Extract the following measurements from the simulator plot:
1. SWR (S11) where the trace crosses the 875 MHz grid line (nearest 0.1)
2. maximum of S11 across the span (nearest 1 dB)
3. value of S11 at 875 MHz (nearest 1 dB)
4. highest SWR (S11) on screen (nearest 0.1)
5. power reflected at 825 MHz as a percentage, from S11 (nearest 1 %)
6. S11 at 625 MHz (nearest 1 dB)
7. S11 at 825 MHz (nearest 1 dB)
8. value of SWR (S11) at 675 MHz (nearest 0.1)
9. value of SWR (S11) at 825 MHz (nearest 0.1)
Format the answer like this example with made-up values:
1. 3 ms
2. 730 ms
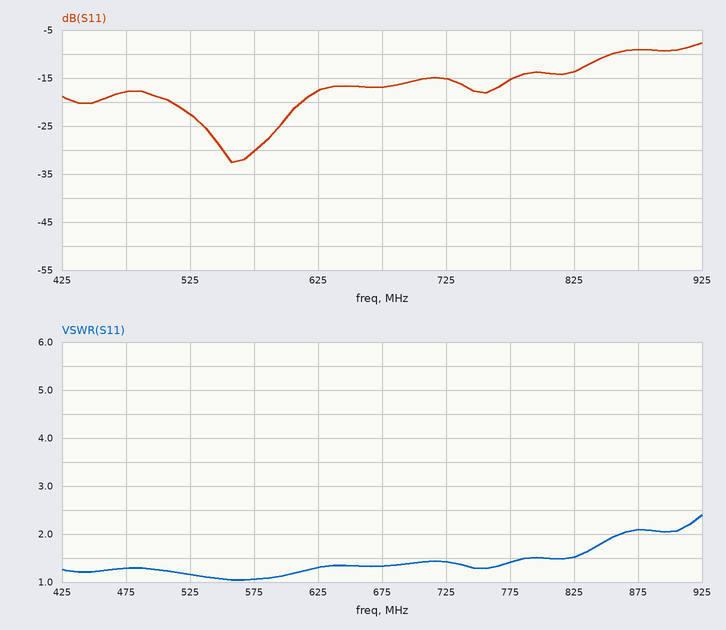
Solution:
1. 2.1
2. -8 dB
3. -9 dB
4. 2.4
5. 4 %
6. -18 dB
7. -14 dB
8. 1.3
9. 1.5
